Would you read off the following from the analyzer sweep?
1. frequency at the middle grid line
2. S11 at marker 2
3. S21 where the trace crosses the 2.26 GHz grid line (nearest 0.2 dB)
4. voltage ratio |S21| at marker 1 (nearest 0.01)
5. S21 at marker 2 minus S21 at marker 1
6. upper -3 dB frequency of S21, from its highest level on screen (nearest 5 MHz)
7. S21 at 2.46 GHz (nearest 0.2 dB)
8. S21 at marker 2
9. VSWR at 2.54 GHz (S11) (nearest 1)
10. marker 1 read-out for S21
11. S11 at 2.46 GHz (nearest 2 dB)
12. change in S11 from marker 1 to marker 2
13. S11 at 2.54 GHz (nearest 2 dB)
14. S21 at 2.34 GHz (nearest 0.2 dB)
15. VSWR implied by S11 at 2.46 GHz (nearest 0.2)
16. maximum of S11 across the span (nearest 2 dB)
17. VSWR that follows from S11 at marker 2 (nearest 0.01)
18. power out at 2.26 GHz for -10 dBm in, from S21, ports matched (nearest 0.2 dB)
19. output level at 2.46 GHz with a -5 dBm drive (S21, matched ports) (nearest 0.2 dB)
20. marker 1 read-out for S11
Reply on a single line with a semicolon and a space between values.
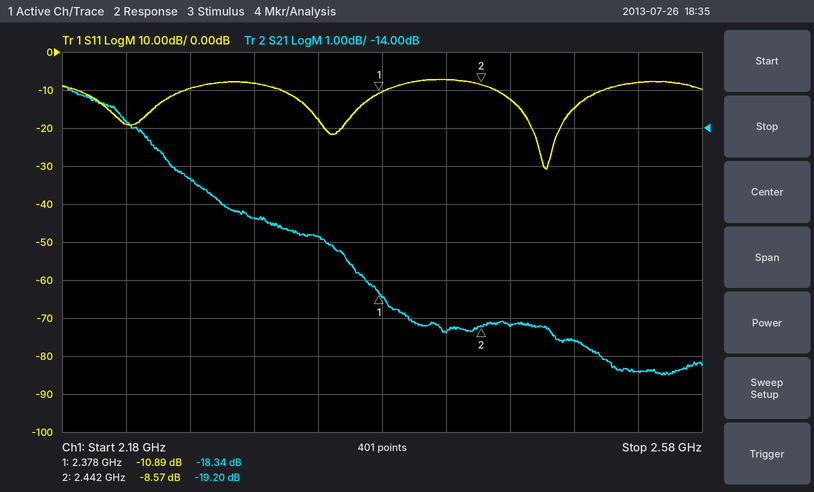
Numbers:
2.38 GHz; -8.57 dB; -15.4 dB; 0.12; -0.86 dB; 2.275 GHz; -19.2 dB; -19.20 dB; 2; -18.34 dB; -12 dB; 2.32 dB; -8 dB; -16.8 dB; 1.6; -8 dB; 2.19; -25.4 dBm; -24.2 dBm; -10.89 dB
